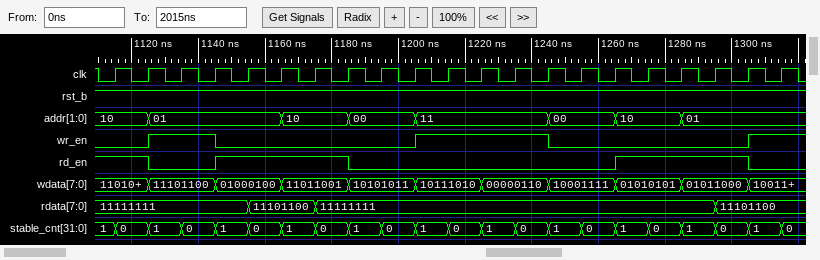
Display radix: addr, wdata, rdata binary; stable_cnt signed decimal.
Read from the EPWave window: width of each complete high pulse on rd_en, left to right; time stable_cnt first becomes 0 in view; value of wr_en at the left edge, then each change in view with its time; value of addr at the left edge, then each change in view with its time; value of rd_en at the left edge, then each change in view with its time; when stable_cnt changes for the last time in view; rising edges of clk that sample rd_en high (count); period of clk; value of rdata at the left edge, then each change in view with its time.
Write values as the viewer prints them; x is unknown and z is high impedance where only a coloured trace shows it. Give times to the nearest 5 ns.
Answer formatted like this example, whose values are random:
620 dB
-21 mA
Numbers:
40 ns, 40 ns
1115 ns
0, 1 at 1125 ns, 0 at 1145 ns, 1 at 1205 ns, 0 at 1245 ns, 1 at 1305 ns
10, 01 at 1125 ns, 10 at 1165 ns, 00 at 1185 ns, 11 at 1205 ns, 00 at 1245 ns, 10 at 1265 ns, 01 at 1285 ns
1, 0 at 1125 ns, 1 at 1145 ns, 0 at 1185 ns, 1 at 1265 ns, 0 at 1305 ns
1315 ns
10
10 ns
11111111, 11101100 at 1155 ns, 11111111 at 1175 ns, 11101100 at 1295 ns
